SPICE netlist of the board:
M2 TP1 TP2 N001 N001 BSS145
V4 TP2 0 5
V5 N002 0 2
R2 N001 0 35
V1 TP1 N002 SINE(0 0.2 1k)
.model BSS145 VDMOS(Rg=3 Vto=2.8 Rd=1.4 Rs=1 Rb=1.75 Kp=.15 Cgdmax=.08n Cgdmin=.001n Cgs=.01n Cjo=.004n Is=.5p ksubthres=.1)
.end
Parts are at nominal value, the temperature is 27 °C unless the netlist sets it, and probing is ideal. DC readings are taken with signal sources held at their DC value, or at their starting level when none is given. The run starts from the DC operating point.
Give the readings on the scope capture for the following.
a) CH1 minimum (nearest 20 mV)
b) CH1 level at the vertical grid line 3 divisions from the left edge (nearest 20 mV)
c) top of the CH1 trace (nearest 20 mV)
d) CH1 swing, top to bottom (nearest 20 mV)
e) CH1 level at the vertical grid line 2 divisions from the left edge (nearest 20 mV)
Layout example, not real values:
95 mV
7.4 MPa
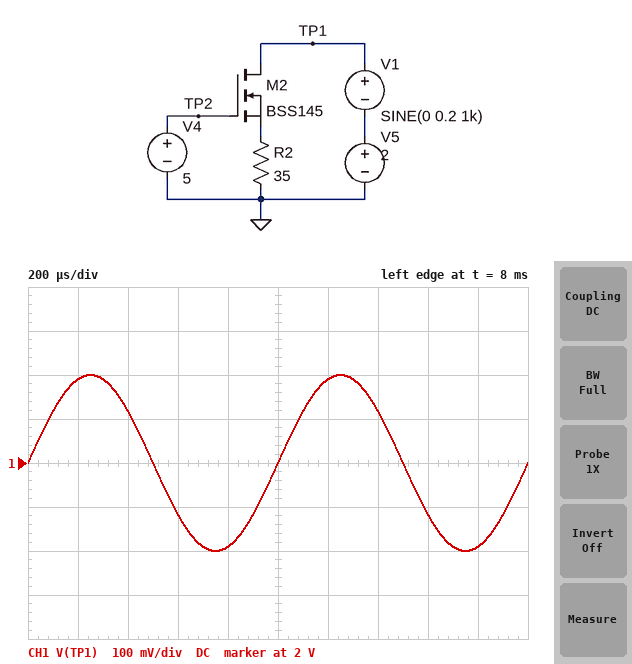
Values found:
1.80 V
1.88 V
2.20 V
400 mV
2.12 V
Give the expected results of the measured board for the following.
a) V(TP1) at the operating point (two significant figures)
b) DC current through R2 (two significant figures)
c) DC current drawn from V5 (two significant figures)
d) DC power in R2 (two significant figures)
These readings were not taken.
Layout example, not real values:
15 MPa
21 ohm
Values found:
2.0 V
40 mA
40 mA
55 mW
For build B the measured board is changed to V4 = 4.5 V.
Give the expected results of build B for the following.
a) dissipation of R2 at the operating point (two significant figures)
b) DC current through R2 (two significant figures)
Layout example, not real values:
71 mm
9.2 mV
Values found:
31 mW
30 mA
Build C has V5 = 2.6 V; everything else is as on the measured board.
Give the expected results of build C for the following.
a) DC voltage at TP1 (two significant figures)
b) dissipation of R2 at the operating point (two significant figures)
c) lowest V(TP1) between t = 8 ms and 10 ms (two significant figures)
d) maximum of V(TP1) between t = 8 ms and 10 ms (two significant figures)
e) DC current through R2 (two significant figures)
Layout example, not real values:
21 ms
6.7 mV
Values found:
2.6 V
58 mW
2.4 V
2.8 V
41 mA
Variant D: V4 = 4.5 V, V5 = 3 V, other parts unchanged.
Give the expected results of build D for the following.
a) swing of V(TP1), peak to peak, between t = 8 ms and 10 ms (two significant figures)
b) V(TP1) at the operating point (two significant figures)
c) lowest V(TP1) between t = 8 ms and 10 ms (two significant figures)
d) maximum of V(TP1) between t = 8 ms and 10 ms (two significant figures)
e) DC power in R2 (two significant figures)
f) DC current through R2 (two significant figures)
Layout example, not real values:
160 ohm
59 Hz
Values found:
400 mV
3.0 V
2.8 V
3.2 V
31 mW
30 mA
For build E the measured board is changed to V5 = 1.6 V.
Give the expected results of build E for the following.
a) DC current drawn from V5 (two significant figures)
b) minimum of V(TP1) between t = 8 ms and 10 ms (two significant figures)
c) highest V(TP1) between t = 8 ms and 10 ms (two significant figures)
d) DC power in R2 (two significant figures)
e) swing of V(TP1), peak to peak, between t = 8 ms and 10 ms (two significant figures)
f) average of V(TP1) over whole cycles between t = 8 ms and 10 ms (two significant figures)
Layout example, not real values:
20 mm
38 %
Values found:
35 mA
1.4 V
1.8 V
43 mW
400 mV
1.6 V
